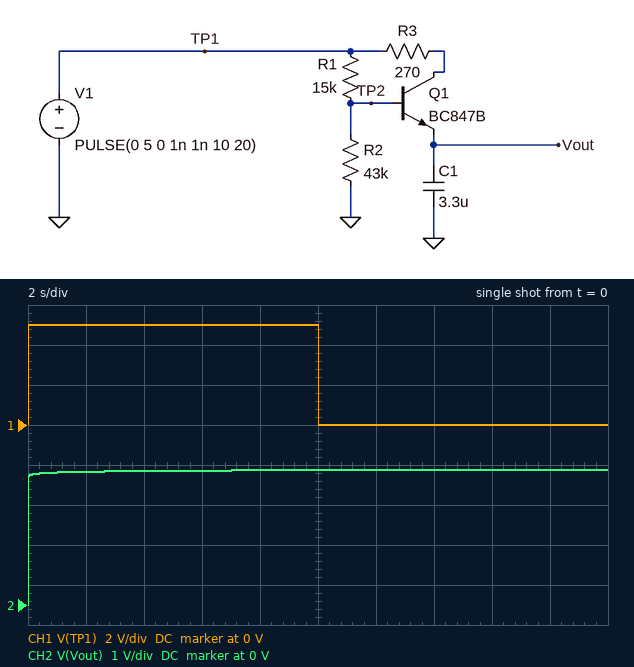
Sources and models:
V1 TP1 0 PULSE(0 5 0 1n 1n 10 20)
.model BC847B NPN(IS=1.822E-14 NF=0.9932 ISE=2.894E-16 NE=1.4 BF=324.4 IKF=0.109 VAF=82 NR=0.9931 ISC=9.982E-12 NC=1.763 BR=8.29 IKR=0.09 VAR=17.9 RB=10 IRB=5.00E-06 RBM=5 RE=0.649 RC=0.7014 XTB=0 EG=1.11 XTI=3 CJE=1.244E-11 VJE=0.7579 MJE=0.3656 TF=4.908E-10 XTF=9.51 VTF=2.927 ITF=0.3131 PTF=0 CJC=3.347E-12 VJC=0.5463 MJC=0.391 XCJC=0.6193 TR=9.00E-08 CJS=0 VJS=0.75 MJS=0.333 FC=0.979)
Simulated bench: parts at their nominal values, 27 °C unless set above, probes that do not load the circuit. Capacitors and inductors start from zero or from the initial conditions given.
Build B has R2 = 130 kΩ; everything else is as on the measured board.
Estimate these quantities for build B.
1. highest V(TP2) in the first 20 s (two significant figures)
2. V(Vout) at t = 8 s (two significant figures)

4.5 V
4.1 V
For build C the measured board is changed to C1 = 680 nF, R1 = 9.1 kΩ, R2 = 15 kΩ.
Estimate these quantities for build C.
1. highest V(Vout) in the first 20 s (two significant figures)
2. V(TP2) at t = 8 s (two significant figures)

2.8 V
3.1 V
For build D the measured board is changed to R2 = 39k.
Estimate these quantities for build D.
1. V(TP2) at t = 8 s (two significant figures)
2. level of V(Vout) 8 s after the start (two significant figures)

3.6 V
3.3 V
